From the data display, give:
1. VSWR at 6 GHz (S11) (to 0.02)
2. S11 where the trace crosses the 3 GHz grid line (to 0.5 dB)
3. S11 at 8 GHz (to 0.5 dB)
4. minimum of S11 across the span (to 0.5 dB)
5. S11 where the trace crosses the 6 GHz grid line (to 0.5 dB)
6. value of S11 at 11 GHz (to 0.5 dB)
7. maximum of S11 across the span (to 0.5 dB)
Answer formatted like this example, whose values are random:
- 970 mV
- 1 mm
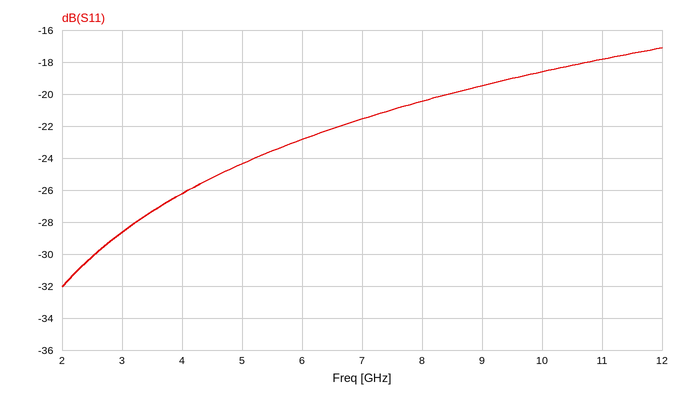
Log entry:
- 1.16
- -28.5 dB
- -20.5 dB
- -32.0 dB
- -23.0 dB
- -18.0 dB
- -17.0 dB
